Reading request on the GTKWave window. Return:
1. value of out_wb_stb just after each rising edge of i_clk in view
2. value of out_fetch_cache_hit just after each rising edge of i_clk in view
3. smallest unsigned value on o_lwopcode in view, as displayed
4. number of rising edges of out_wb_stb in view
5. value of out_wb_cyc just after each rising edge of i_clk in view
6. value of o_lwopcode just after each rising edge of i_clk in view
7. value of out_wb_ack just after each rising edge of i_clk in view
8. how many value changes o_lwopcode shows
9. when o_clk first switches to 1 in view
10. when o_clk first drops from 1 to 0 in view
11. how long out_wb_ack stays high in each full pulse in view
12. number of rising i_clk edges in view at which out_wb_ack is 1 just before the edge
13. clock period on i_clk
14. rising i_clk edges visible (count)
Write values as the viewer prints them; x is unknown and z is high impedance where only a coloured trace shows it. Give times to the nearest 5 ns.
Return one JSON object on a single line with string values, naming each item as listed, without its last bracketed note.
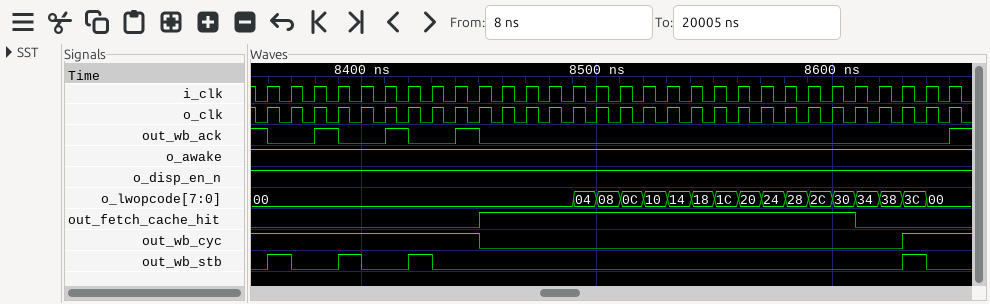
{"value of out_wb_stb just after each rising edge of i_clk in view": "1 0 0 1 0 0 1 0 0 0 0 0 0 0 0 0 0 0 0 0 0 0 0 0 0 0 0 1 0 0", "value of out_fetch_cache_hit just after each rising edge of i_clk in view": "0 0 0 0 0 0 0 0 0 1 1 1 1 1 1 1 1 1 1 1 1 1 1 1 1 0 0 0 0 0", "smallest unsigned value on o_lwopcode in view, as displayed": "00", "number of rising edges of out_wb_stb in view": "4", "value of out_wb_cyc just after each rising edge of i_clk in view": "1 1 1 1 1 1 1 1 1 0 0 0 0 0 0 0 0 0 0 0 0 0 0 0 0 0 0 1 1 1", "value of o_lwopcode just after each rising edge of i_clk in view": "00, 00, 00, 00, 00, 00, 00, 00, 00, 00, 00, 00, 00, 04, 08, 0C, 10, 14, 18, 1C, 20, 24, 28, 2C, 30, 34, 38, 3C, 00, 00", "value of out_wb_ack just after each rising edge of i_clk in view": "0 0 1 0 0 1 0 0 1 0 0 0 0 0 0 0 0 0 0 0 0 0 0 0 0 0 0 0 0 1", "how many value changes o_lwopcode shows": "16", "when o_clk first switches to 1 in view": "8360 ns", "when o_clk first drops from 1 to 0 in view": "8355 ns", "how long out_wb_ack stays high in each full pulse in view": "10 ns, 10 ns, 10 ns", "number of rising i_clk edges in view at which out_wb_ack is 1 just before the edge": "4", "clock period on i_clk": "10 ns", "rising i_clk edges visible": "30"}
